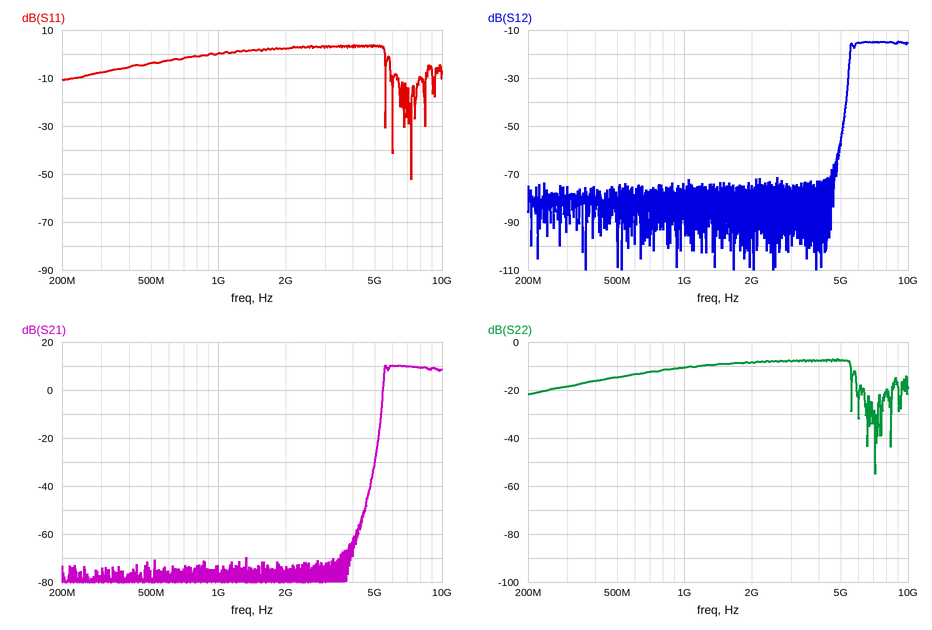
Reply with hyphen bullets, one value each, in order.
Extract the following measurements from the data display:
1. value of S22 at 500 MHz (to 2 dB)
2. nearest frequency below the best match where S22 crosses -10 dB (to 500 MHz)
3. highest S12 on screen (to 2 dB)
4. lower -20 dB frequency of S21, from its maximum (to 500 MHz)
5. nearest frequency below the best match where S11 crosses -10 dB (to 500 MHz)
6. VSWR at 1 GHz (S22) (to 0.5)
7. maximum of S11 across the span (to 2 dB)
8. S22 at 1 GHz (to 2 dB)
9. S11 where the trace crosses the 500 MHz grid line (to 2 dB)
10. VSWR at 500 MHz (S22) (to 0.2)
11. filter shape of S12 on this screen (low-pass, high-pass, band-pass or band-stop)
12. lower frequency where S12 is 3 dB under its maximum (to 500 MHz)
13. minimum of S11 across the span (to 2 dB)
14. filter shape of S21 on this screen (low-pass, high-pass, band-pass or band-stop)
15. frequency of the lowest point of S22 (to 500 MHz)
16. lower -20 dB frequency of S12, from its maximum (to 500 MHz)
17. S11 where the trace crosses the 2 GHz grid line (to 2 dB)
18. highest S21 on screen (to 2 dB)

- -14 dB
- 5.5 GHz
- -14 dB
- 5.5 GHz
- 6.5 GHz
- 2.0
- 4 dB
- -10 dB
- -4 dB
- 1.4
- high-pass
- 5.5 GHz
- -52 dB
- high-pass
- 7.0 GHz
- 5.5 GHz
- 2 dB
- 10 dB
